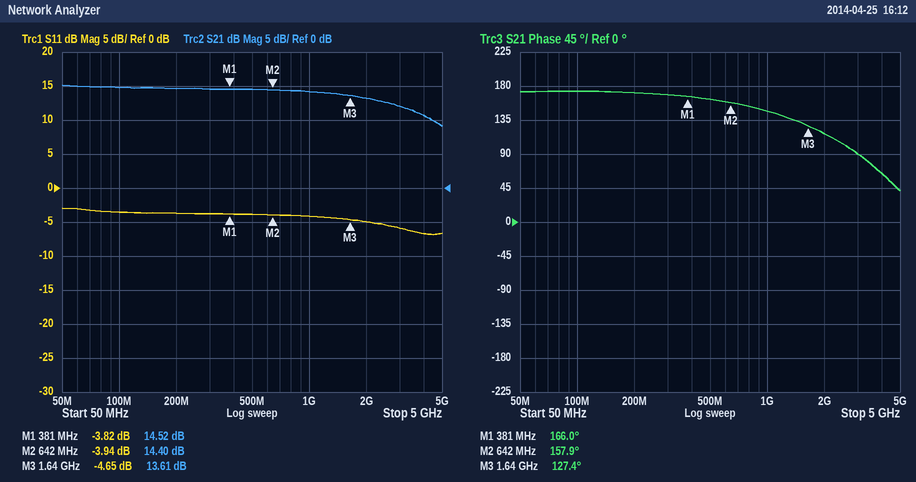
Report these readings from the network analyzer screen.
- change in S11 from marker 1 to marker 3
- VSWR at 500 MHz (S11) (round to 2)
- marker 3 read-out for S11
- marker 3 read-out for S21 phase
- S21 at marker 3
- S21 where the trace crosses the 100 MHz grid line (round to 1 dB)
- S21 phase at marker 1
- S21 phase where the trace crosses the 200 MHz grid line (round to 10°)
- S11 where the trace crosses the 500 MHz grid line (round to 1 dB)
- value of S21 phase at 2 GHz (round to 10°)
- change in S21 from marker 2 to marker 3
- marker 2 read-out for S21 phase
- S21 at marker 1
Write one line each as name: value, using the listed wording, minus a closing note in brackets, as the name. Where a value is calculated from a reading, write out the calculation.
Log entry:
change in S11 from marker 1 to marker 3: -4.65 − (-3.82) = -0.83 dB
VSWR at 500 MHz (S11): |Γ| = 10^(-4/20) = 0.6310; VSWR = (1 + 0.6310)/(1 − 0.6310) ≈ 4
marker 3 read-out for S11: -4.65 dB
marker 3 read-out for S21 phase: 127.4°
S21 at marker 3: 13.61 dB
S21 where the trace crosses the 100 MHz grid line: 15 dB
S21 phase at marker 1: 166.0°
S21 phase where the trace crosses the 200 MHz grid line: 170°
S11 where the trace crosses the 500 MHz grid line: -4 dB
value of S21 phase at 2 GHz: 120°
change in S21 from marker 2 to marker 3: 13.61 − (14.4) = -0.79 dB
marker 2 read-out for S21 phase: 157.9°
S21 at marker 1: 14.52 dB
